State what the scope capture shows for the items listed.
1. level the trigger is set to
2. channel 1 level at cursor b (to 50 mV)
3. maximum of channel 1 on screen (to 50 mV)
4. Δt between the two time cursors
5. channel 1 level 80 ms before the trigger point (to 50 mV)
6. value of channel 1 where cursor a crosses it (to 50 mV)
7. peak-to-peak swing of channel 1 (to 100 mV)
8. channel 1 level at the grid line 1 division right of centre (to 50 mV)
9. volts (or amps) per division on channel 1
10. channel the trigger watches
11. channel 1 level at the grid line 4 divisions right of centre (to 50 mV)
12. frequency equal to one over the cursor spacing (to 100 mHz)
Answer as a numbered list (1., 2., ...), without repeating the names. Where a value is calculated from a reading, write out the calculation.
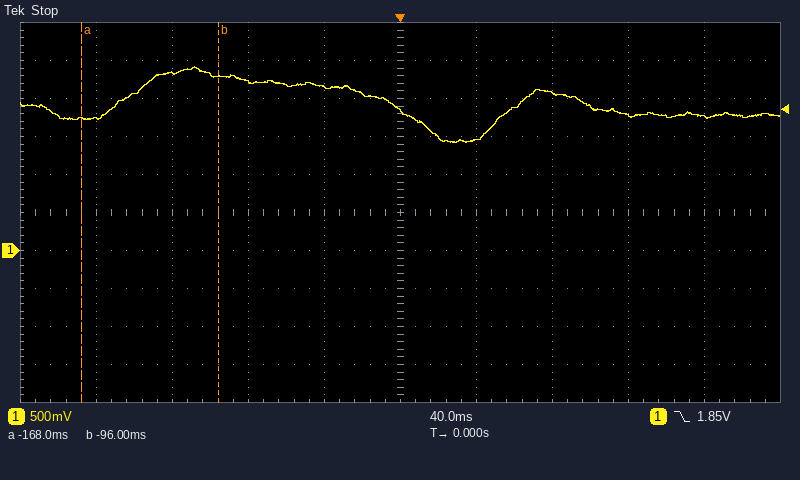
1. 1.85 V
2. 2.30 V
3. 2.40 V
4. -96 ms − (-168 ms) = 72 ms
5. 2.20 V
6. 1.75 V
7. 1.00 V
8. 1.45 V
9. 500 mV
10. channel 1
11. 1.75 V
12. 1 / 72 ms ≈ 13.9 Hz
